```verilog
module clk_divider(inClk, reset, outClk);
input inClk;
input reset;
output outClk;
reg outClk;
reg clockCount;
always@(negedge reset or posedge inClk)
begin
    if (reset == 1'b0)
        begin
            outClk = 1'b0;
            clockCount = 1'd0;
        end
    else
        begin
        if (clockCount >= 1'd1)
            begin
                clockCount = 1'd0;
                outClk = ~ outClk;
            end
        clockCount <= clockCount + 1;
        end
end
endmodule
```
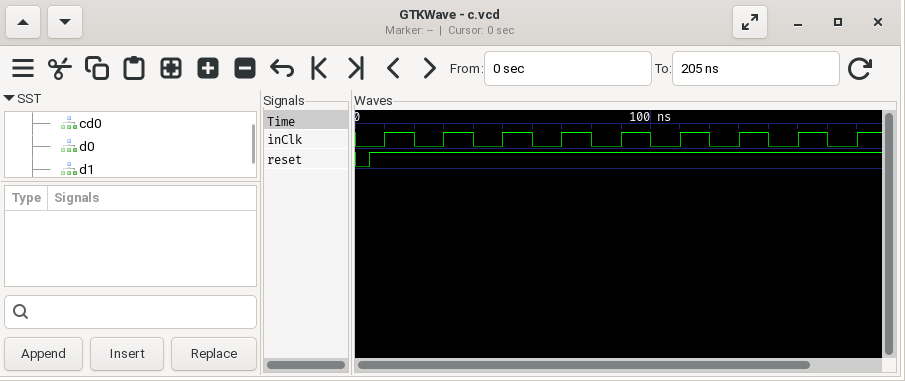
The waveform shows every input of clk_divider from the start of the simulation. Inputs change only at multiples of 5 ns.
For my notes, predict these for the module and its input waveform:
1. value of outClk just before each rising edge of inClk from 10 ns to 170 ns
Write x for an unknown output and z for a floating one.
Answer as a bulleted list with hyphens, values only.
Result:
- 0 0 1 0 1 0 1 0 1
